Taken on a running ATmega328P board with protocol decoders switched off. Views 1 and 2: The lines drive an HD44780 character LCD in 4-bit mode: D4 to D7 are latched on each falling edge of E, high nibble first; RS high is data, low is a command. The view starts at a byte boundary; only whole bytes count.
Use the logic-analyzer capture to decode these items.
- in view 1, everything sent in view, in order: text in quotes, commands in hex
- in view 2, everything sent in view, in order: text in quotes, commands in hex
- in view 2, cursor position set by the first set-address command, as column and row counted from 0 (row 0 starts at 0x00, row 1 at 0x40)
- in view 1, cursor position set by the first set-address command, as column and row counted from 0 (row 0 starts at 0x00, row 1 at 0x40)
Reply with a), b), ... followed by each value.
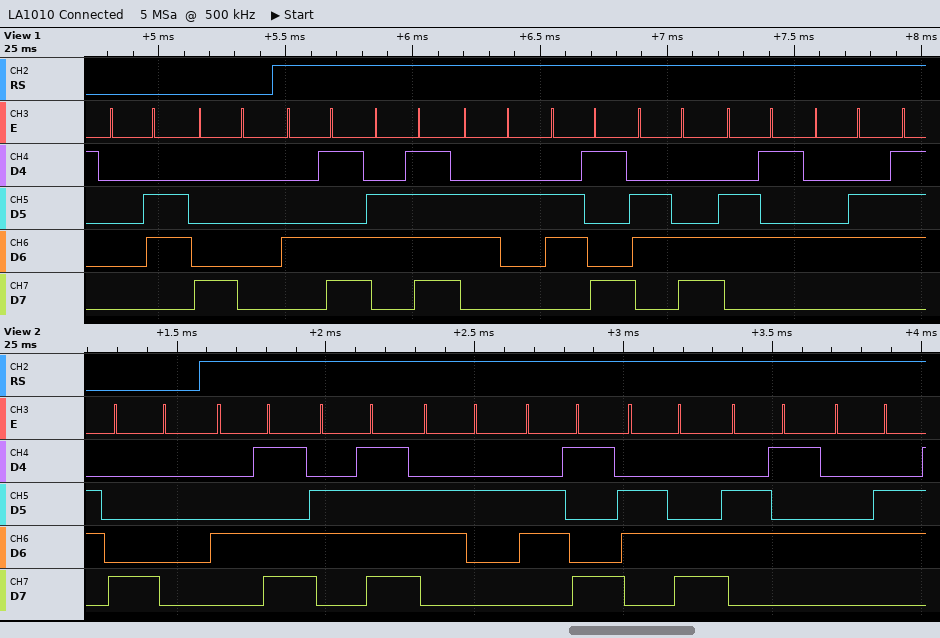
a) 0x06 0x80 "MobileF"
b) 0x80 "MobileF"
c) column 0, row 0
d) column 0, row 0
